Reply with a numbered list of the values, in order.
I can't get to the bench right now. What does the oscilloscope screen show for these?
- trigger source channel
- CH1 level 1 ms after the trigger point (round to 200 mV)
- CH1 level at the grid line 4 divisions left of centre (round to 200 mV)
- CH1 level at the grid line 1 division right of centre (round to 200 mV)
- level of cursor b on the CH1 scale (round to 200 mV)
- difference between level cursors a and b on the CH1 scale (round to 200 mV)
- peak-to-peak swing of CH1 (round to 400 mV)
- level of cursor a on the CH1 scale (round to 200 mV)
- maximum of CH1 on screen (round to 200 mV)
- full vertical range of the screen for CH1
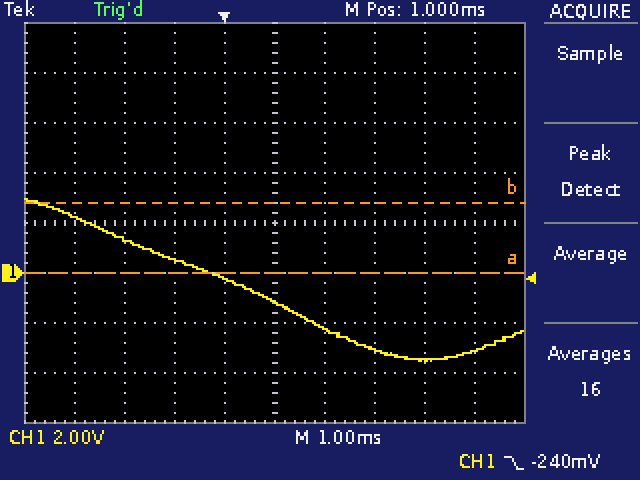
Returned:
1. CH1
2. -1.2 V
3. 2.2 V
4. -2.2 V
5. 2.8 V
6. 2.8 V
7. 6.4 V
8. 0.0 V
9. 3.0 V
10. 16 V
